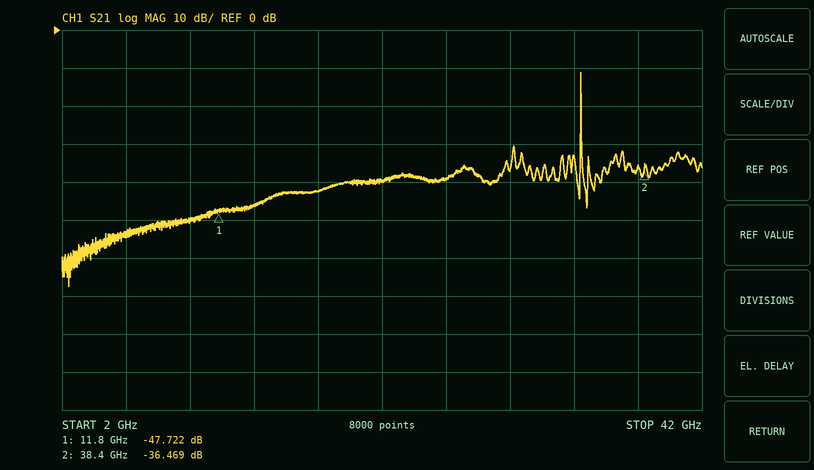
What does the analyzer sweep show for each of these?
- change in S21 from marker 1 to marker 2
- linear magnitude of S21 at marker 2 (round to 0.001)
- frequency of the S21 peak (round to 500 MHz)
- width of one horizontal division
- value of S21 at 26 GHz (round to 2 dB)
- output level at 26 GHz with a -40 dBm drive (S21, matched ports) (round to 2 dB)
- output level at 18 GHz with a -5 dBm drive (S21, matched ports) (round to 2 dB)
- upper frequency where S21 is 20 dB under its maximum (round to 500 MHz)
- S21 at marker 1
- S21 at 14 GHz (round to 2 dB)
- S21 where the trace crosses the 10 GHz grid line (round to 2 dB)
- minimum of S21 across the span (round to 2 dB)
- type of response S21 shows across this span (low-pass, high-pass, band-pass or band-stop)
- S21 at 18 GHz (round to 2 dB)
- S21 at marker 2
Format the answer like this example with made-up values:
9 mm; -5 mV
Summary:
11.253 dB; 0.015; 34.5 GHz; 4 GHz; -40 dB; -80 dBm; -48 dBm; 34.5 GHz; -47.722 dB; -46 dB; -50 dB; -68 dB; band-pass; -42 dB; -36.469 dB
